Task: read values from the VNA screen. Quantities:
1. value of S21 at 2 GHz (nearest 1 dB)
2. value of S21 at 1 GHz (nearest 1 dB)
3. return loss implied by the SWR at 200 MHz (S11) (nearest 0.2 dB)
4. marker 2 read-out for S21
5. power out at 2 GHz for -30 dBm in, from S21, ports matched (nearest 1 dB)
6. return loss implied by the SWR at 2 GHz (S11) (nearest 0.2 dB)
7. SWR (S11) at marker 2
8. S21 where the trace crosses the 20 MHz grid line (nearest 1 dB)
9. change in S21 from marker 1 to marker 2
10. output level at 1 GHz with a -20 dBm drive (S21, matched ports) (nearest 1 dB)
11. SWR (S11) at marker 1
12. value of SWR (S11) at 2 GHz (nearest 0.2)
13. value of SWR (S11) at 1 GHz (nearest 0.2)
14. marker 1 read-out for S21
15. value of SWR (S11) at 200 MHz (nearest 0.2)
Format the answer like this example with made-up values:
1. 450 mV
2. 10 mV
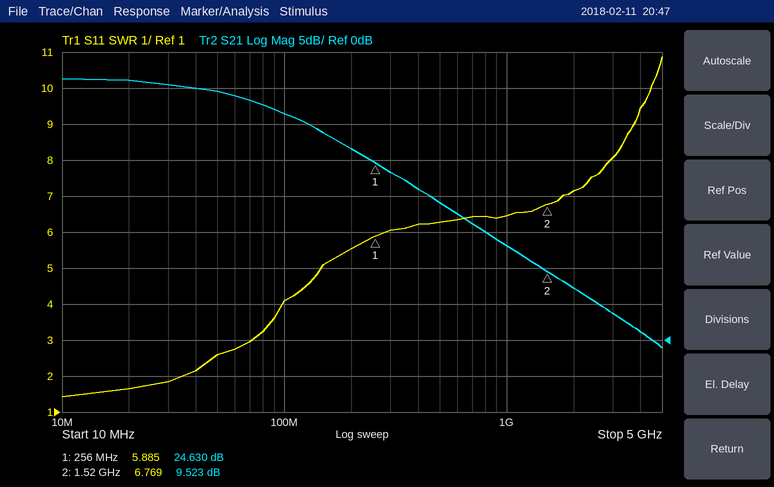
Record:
1. 7 dB
2. 13 dB
3. 3.2 dB
4. 9.523 dB
5. -23 dBm
6. 2.4 dB
7. 6.769
8. 36 dB
9. -15.107 dB
10. -7 dBm
11. 5.885
12. 7.2
13. 6.4
14. 24.630 dB
15. 5.6
